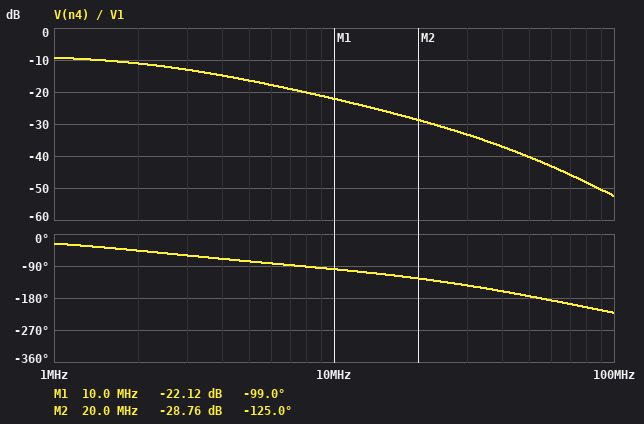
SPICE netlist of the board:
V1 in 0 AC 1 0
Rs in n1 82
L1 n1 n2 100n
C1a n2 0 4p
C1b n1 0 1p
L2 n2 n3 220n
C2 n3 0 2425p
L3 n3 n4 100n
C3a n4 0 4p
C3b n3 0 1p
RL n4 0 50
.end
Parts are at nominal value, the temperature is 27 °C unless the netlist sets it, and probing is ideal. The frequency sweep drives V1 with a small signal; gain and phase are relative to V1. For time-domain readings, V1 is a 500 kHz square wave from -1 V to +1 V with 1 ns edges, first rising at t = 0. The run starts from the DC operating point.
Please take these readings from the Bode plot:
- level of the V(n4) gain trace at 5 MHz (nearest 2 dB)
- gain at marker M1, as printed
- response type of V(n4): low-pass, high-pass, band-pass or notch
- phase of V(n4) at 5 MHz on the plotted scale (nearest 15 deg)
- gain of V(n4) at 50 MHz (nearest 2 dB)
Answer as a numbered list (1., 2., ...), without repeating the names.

1. -16 dB
2. -22.12 dB
3. low-pass
4. -75 deg
5. -40 dB
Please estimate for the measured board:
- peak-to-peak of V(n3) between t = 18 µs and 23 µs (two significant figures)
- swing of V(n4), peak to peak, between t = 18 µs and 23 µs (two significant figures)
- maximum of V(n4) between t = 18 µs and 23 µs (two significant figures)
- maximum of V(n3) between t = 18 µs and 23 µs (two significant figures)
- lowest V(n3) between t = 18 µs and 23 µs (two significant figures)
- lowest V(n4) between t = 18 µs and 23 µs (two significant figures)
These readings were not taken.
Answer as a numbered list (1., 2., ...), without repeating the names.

1. 760 mV
2. 760 mV
3. 380 mV
4. 380 mV
5. -380 mV
6. -380 mV
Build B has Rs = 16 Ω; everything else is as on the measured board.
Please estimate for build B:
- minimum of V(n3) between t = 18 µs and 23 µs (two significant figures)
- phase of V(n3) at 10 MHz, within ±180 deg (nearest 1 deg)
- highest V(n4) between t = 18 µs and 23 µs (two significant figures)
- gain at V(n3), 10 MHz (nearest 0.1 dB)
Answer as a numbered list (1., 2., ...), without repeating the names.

1. -830 mV
2. -121 deg
3. 830 mV
4. -10.3 dB
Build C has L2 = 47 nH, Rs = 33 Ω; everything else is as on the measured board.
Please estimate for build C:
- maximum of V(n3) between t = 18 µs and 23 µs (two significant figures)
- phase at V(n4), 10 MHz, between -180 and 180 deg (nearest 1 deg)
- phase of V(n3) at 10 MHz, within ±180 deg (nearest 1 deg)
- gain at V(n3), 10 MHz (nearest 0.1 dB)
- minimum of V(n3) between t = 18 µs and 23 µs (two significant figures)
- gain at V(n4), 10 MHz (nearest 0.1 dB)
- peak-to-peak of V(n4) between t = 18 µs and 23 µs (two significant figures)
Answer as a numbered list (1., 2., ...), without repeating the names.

1. 600 mV
2. -94 deg
3. -87 deg
4. -14.2 dB
5. -600 mV
6. -14.3 dB
7. 1.2 V
